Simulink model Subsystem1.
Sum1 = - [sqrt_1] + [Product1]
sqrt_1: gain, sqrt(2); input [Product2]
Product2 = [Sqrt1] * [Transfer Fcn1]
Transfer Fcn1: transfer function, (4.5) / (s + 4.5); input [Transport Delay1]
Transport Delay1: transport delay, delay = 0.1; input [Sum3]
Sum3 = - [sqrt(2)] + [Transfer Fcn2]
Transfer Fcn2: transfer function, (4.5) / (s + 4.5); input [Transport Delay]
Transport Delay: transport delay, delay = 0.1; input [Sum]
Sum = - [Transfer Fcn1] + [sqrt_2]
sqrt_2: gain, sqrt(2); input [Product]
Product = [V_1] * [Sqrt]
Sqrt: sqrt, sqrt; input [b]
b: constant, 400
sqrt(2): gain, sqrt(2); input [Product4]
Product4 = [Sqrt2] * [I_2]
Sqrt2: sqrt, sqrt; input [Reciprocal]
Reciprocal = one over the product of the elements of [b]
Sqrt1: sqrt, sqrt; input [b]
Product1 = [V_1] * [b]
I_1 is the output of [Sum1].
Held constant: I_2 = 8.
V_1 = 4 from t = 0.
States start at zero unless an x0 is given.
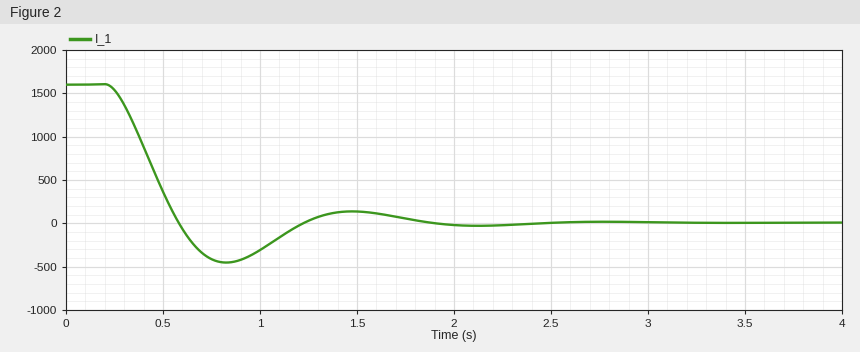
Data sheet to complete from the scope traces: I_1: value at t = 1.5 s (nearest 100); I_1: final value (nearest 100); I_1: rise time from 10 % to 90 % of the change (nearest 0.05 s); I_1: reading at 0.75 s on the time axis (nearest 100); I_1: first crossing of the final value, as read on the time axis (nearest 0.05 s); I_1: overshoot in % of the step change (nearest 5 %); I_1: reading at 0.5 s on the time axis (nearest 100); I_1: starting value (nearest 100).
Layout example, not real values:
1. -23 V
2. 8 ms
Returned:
1. 100
2. 0
3. 0.25 s
4. -400
5. 0.60 s
6. 30 %
7. 400
8. 1600
